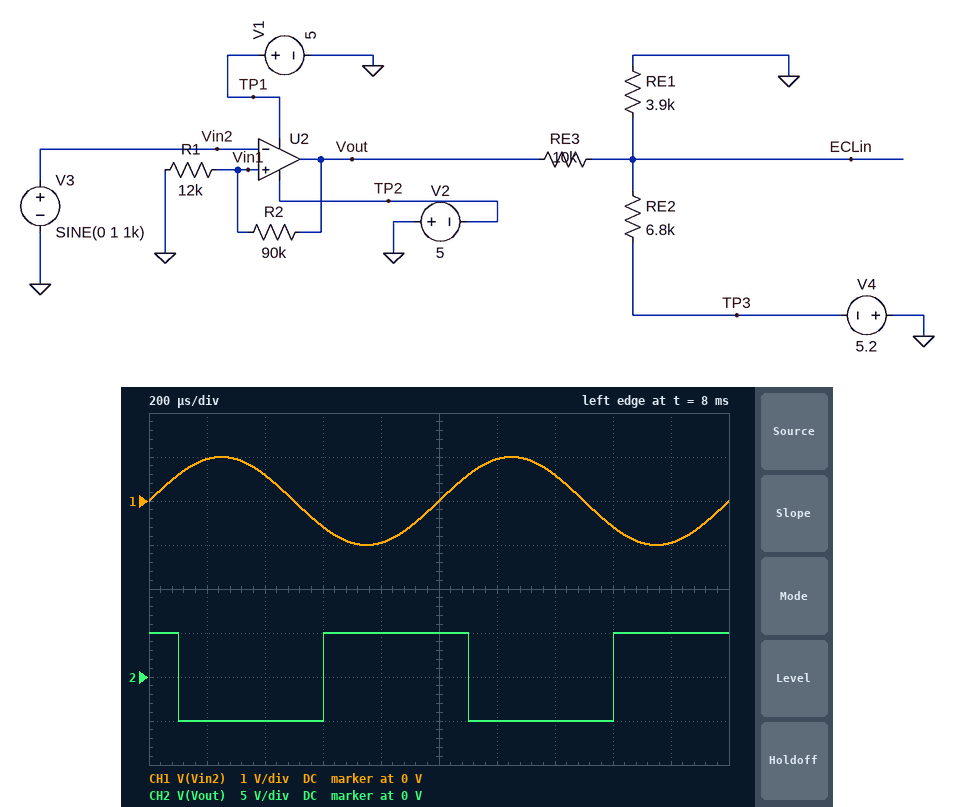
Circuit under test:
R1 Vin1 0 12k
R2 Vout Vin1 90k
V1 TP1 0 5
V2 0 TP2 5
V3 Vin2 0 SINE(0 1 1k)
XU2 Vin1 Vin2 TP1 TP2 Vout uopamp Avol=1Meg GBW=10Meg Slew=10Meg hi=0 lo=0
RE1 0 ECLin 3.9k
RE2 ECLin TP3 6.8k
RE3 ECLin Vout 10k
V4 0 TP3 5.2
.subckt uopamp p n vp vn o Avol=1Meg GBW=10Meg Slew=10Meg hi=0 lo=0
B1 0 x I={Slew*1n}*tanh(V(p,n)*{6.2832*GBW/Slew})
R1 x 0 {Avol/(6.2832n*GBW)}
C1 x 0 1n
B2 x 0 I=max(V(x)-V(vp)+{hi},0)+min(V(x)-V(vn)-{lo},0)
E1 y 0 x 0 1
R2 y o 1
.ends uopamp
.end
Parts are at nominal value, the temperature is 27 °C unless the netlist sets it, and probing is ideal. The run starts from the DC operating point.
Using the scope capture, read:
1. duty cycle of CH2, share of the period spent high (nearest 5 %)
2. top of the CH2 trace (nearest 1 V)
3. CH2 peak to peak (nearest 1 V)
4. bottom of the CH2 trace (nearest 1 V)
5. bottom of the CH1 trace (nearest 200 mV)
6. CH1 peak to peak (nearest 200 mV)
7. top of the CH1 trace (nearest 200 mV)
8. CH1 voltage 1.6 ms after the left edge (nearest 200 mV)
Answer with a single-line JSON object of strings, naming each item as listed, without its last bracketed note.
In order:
{"duty cycle of CH2, share of the period spent high": "50 %", "top of the CH2 trace": "5 V", "CH2 peak to peak": "10 V", "bottom of the CH2 trace": "-5 V", "bottom of the CH1 trace": "-1.0 V", "CH1 peak to peak": "2.0 V", "top of the CH1 trace": "1.0 V", "CH1 voltage 1.6 ms after the left edge": "-600 mV"}
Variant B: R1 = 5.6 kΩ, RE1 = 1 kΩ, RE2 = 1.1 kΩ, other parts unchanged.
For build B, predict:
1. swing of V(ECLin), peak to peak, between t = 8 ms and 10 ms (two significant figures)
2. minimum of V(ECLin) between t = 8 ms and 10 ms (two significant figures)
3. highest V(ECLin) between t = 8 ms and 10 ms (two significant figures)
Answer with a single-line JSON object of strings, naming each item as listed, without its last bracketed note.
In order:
{"swing of V(ECLin), peak to peak, between t = 8 ms and 10 ms": "500 mV", "minimum of V(ECLin) between t = 8 ms and 10 ms": "-2.6 V", "highest V(ECLin) between t = 8 ms and 10 ms": "-2.1 V"}
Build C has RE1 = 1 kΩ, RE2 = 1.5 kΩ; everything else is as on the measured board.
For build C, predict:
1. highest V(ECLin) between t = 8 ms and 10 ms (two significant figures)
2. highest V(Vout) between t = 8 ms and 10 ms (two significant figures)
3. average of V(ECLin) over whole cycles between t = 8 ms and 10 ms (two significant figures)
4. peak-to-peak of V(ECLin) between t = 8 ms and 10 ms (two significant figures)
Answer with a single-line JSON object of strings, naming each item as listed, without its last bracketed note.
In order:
{"highest V(ECLin) between t = 8 ms and 10 ms": "-1.7 V", "highest V(Vout) between t = 8 ms and 10 ms": "5.0 V", "average of V(ECLin) over whole cycles between t = 8 ms and 10 ms": "-2.0 V", "peak-to-peak of V(ECLin) between t = 8 ms and 10 ms": "570 mV"}
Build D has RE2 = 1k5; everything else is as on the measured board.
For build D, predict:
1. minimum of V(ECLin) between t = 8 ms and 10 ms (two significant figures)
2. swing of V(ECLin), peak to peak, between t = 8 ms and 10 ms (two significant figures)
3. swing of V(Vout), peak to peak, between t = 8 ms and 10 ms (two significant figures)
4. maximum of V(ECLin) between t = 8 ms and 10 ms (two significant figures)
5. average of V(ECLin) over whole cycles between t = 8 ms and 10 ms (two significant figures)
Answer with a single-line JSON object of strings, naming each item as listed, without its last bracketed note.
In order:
{"minimum of V(ECLin) between t = 8 ms and 10 ms": "-3.9 V", "swing of V(ECLin), peak to peak, between t = 8 ms and 10 ms": "980 mV", "swing of V(Vout), peak to peak, between t = 8 ms and 10 ms": "10 V", "maximum of V(ECLin) between t = 8 ms and 10 ms": "-2.9 V", "average of V(ECLin) over whole cycles between t = 8 ms and 10 ms": "-3.4 V"}
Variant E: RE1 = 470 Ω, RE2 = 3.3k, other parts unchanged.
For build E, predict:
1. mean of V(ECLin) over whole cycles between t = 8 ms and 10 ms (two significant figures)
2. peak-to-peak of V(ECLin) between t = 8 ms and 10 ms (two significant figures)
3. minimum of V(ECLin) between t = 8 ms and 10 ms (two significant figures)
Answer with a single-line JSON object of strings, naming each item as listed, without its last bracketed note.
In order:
{"mean of V(ECLin) over whole cycles between t = 8 ms and 10 ms": "-620 mV", "peak-to-peak of V(ECLin) between t = 8 ms and 10 ms": "400 mV", "minimum of V(ECLin) between t = 8 ms and 10 ms": "-820 mV"}
